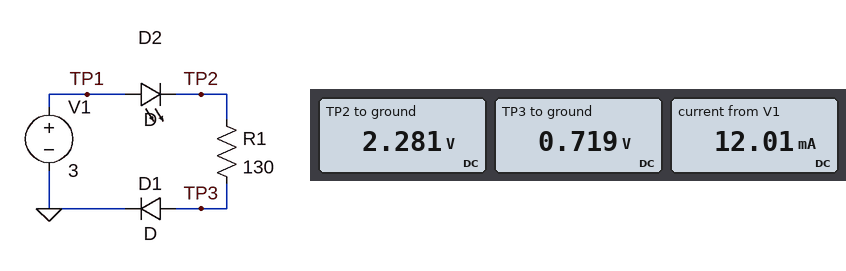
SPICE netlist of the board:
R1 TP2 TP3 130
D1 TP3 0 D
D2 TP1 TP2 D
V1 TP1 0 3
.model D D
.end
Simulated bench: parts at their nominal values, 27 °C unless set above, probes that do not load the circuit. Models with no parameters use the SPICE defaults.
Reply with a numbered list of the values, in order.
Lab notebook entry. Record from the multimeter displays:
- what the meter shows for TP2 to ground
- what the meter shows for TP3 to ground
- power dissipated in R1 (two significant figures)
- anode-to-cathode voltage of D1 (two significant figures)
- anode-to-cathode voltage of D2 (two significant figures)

1. 2.281 V
2. 0.719 V
3. 19 mW
4. 720 mV
5. 720 mV
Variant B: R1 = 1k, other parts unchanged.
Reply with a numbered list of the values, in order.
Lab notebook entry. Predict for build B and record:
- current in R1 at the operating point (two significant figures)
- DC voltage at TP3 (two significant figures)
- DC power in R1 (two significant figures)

1. 1.7 mA
2. 670 mV
3. 2.8 mW
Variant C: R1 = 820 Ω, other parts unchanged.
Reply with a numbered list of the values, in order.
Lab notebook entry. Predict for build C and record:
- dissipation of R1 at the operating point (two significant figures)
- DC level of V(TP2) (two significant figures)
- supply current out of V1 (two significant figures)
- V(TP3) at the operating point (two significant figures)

1. 3.3 mW
2. 2.3 V
3. 2.0 mA
4. 670 mV
